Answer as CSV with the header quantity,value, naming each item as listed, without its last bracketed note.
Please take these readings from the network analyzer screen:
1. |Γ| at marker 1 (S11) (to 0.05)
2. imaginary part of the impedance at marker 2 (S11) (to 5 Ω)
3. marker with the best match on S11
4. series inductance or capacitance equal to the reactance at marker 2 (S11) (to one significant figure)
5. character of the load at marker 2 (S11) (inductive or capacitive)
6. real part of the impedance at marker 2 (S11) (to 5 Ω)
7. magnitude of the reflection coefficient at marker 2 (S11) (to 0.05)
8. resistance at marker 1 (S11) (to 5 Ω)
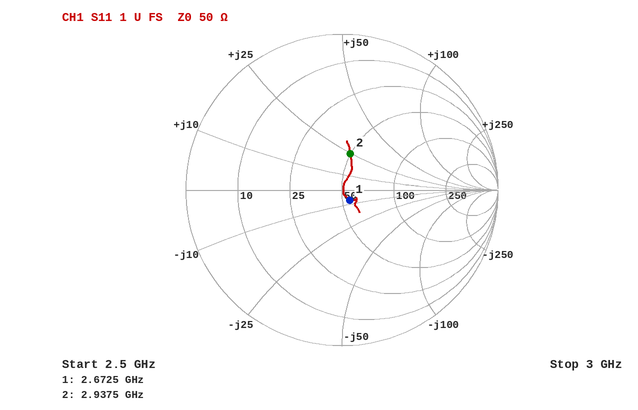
quantity,value
|Γ| at marker 1 (S11),0.10
imaginary part of the impedance at marker 2 (S11),+25 Ω
marker with the best match on S11,marker 1
series inductance or capacitance equal to the reactance at marker 2 (S11),1 nH
character of the load at marker 2 (S11),inductive
real part of the impedance at marker 2 (S11),50 Ω
magnitude of the reflection coefficient at marker 2 (S11),0.25
resistance at marker 1 (S11),55 Ω
